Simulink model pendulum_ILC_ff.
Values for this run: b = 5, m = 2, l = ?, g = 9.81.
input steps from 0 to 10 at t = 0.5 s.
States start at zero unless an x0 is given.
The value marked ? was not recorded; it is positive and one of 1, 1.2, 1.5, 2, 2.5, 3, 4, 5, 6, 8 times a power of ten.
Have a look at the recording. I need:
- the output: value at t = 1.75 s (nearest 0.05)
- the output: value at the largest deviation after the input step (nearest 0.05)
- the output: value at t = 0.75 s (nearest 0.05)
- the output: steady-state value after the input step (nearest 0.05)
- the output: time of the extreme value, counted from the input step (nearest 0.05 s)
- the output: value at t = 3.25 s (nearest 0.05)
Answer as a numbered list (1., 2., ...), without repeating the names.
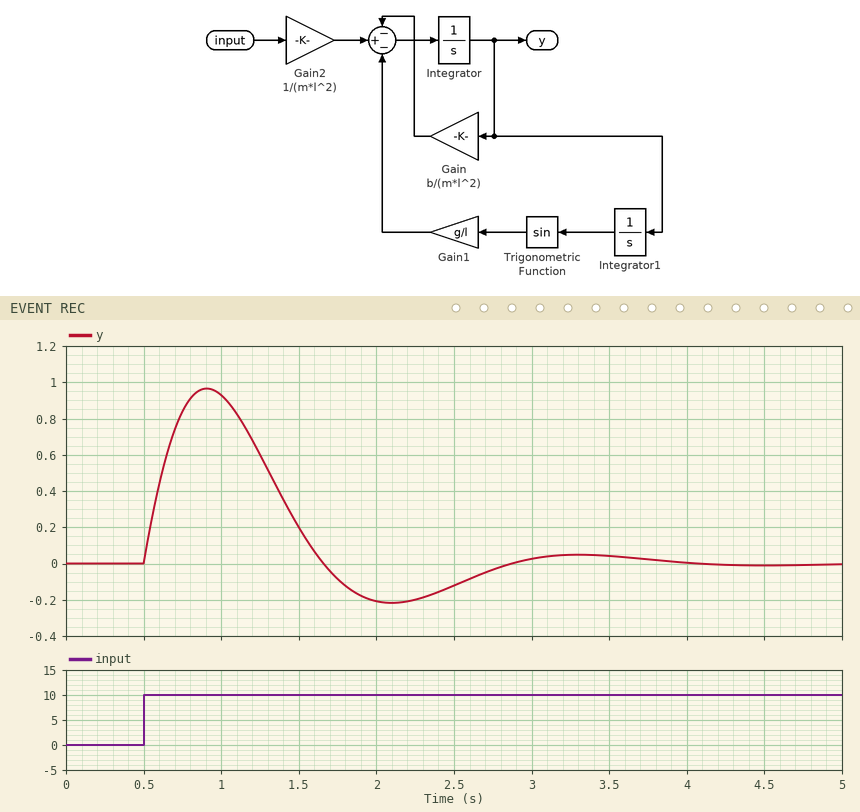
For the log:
1. -0.10
2. 0.95
3. 0.85
4. 0.00
5. 0.40 s
6. 0.05
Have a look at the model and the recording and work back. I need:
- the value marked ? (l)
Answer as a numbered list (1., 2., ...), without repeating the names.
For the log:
1. 1
